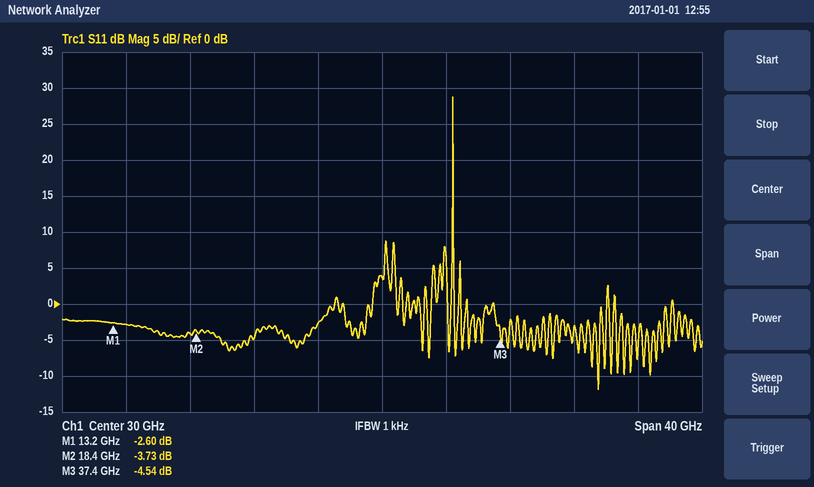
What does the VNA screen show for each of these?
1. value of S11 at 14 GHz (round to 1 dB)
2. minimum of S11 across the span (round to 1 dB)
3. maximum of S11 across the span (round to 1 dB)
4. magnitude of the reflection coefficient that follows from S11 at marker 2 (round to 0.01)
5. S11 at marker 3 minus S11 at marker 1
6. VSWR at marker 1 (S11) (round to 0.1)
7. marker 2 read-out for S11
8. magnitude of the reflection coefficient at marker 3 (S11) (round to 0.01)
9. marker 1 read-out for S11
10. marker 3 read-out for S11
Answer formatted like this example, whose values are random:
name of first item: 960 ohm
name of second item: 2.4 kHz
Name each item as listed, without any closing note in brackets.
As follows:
value of S11 at 14 GHz: -3 dB
minimum of S11 across the span: -12 dB
maximum of S11 across the span: 29 dB
magnitude of the reflection coefficient that follows from S11 at marker 2: 0.65
S11 at marker 3 minus S11 at marker 1: -1.94 dB
VSWR at marker 1 (S11): 6.7
marker 2 read-out for S11: -3.73 dB
magnitude of the reflection coefficient at marker 3 (S11): 0.59
marker 1 read-out for S11: -2.60 dB
marker 3 read-out for S11: -4.54 dB
